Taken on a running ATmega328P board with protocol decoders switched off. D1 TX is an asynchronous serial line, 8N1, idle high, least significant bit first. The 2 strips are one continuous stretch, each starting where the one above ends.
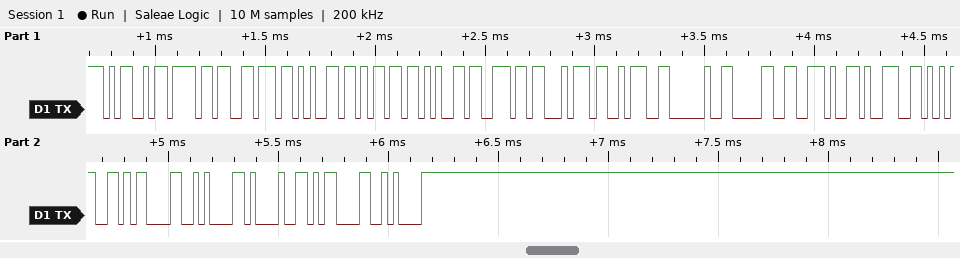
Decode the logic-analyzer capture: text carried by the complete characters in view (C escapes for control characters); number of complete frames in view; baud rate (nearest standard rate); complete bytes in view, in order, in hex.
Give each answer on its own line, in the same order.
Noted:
"Movement: 0.95\r\n!\r\n"
19
38400 baud
4D 6F 76 65 6D 65 6E 74 3A 20 30 2E 39 35 0D 0A 21 0D 0A
